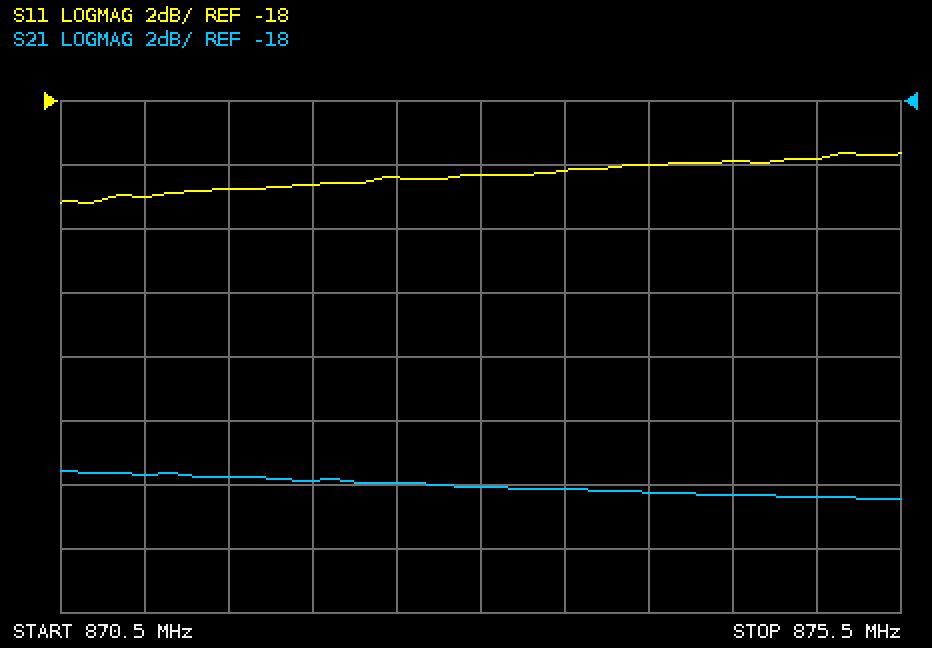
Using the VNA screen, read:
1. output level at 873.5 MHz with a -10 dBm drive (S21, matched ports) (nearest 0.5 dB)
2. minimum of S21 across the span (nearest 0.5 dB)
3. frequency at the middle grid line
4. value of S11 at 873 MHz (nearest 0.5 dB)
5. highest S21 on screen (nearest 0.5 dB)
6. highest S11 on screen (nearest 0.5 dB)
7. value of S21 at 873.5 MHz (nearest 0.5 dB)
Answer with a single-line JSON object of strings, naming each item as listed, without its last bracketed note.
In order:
{"output level at 873.5 MHz with a -10 dBm drive (S21, matched ports)": "-40.0 dBm", "minimum of S21 across the span": "-30.5 dB", "frequency at the middle grid line": "873 MHz", "value of S11 at 873 MHz": "-20.5 dB", "highest S21 on screen": "-29.5 dB", "highest S11 on screen": "-19.5 dB", "value of S21 at 873.5 MHz": "-30.0 dB"}
